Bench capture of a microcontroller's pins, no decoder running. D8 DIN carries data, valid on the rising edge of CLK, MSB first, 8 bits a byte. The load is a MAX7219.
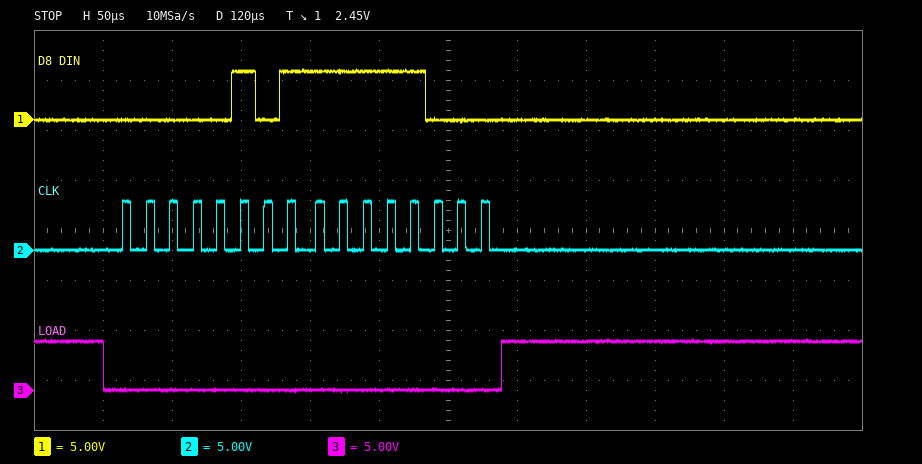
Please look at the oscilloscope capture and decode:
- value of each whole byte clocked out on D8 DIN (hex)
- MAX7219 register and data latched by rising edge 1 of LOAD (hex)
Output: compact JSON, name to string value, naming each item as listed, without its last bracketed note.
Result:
{"value of each whole byte clocked out on D8 DIN": "05 F8", "MAX7219 register and data latched by rising edge 1 of LOAD": "register 0x5, data 0xF8"}
